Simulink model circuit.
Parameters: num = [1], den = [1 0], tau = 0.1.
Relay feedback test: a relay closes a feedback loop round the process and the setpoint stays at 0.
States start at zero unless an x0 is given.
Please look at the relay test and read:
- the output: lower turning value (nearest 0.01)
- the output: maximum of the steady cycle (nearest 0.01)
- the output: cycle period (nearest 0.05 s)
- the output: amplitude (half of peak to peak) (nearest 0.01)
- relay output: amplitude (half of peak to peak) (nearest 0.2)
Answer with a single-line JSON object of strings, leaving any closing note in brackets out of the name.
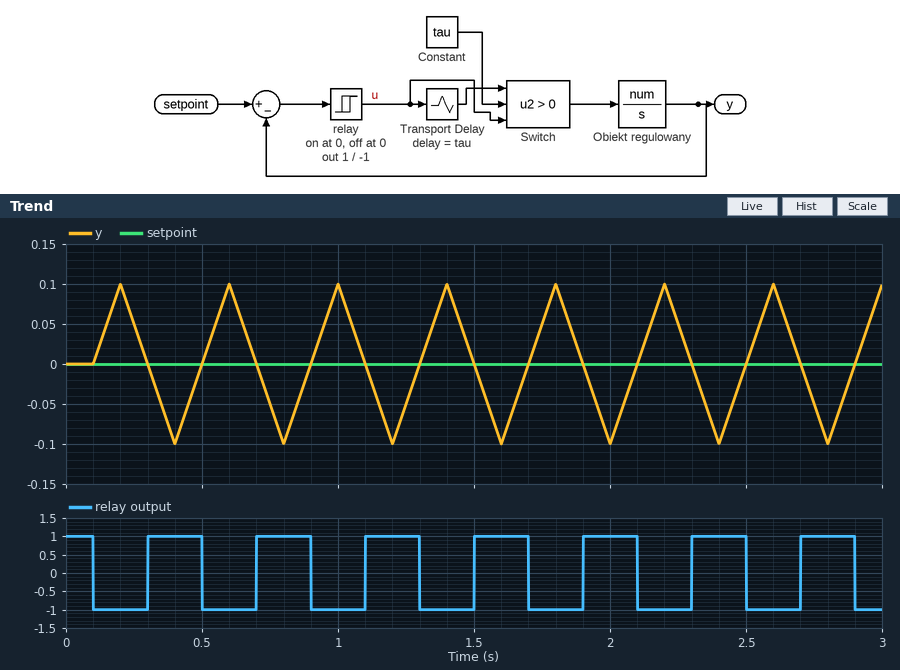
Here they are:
{"the output: lower turning value": "-0.10", "the output: maximum of the steady cycle": "0.10", "the output: cycle period": "0.40 s", "the output: amplitude (half of peak to peak)": "0.10", "relay output: amplitude (half of peak to peak)": "1.0"}
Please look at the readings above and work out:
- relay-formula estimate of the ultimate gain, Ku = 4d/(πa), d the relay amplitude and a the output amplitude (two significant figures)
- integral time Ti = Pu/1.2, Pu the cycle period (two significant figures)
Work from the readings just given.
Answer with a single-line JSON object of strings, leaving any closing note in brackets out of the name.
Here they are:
{"relay-formula estimate of the ultimate gain, Ku = 4d/(πa), d the relay amplitude and a the output amplitude": "13", "integral time Ti = Pu/1.2, Pu the cycle period": "0.33 s"}
